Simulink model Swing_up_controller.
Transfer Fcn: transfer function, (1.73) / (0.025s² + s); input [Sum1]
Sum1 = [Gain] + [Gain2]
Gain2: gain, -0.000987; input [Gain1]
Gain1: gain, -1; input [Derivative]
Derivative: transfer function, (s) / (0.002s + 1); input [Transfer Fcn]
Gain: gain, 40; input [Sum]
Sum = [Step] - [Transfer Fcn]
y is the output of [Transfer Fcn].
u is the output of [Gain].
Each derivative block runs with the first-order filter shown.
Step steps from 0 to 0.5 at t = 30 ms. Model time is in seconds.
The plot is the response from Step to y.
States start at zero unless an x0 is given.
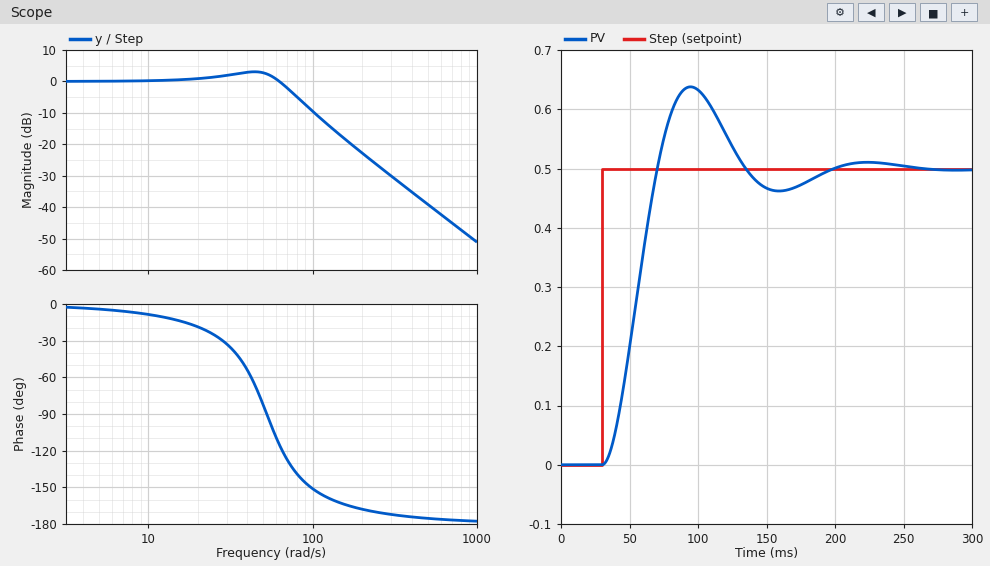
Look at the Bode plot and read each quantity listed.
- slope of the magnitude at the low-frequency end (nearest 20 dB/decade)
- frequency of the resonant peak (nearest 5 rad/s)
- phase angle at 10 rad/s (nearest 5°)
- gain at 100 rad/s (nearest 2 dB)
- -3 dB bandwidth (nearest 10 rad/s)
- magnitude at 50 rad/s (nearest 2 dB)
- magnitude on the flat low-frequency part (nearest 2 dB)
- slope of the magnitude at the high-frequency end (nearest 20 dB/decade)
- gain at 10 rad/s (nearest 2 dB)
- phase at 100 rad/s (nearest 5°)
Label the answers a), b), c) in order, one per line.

a) 0 dB/decade
b) 45 rad/s
c) -10°
d) -10 dB
e) 70 rad/s
f) 2 dB
g) 0 dB
h) -40 dB/decade
i) 0 dB
j) -150°
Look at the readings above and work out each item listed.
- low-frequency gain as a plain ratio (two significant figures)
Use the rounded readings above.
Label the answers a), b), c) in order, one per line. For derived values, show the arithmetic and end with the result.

a) 10^(0 / 20) = 1.0
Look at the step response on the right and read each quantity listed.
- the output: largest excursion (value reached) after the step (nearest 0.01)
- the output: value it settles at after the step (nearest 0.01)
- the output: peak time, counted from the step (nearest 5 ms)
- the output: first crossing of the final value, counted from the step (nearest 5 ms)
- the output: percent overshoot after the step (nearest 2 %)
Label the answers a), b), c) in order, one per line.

a) 0.64
b) 0.50
c) 65 ms
d) 40 ms
e) 28 %
